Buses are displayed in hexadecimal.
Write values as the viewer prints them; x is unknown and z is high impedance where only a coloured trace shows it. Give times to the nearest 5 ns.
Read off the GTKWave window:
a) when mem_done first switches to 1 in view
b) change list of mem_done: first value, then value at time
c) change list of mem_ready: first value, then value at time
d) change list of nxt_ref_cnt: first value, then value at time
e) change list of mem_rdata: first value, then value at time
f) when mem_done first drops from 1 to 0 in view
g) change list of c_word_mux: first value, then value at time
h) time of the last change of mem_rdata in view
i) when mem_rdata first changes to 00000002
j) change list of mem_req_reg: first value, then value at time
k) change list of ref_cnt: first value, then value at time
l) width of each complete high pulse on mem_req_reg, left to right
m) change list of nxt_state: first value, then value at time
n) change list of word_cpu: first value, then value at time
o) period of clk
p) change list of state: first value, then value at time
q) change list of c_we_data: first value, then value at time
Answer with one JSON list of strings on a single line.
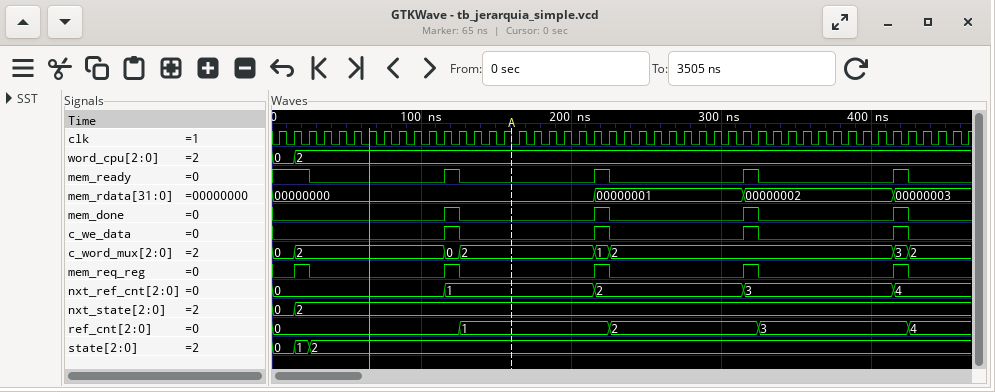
["115 ns", "0, 1 at 115 ns, 0 at 125 ns, 1 at 215 ns, 0 at 225 ns, 1 at 315 ns, 0 at 325 ns, 1 at 415 ns, 0 at 425 ns", "1, 0 at 25 ns, 1 at 115 ns, 0 at 125 ns, 1 at 215 ns, 0 at 225 ns, 1 at 315 ns, 0 at 325 ns, 1 at 415 ns, 0 at 425 ns", "0, 1 at 115 ns, 2 at 215 ns, 3 at 315 ns, 4 at 415 ns", "00000000, 00000001 at 215 ns, 00000002 at 315 ns, 00000003 at 415 ns", "125 ns", "0, 2 at 15 ns, 0 at 115 ns, 2 at 125 ns, 1 at 215 ns, 2 at 225 ns, 3 at 415 ns, 2 at 425 ns", "415 ns", "315 ns", "0, 1 at 15 ns, 0 at 25 ns, 1 at 115 ns, 0 at 125 ns, 1 at 215 ns, 0 at 225 ns, 1 at 315 ns, 0 at 325 ns, 1 at 415 ns, 0 at 425 ns", "0, 1 at 125 ns, 2 at 225 ns, 3 at 325 ns, 4 at 425 ns", "10 ns, 10 ns, 10 ns, 10 ns, 10 ns", "0, 2 at 15 ns", "0, 2 at 15 ns", "10 ns", "0, 1 at 15 ns, 2 at 25 ns", "0, 1 at 115 ns, 0 at 125 ns, 1 at 215 ns, 0 at 225 ns, 1 at 315 ns, 0 at 325 ns, 1 at 415 ns, 0 at 425 ns"]
